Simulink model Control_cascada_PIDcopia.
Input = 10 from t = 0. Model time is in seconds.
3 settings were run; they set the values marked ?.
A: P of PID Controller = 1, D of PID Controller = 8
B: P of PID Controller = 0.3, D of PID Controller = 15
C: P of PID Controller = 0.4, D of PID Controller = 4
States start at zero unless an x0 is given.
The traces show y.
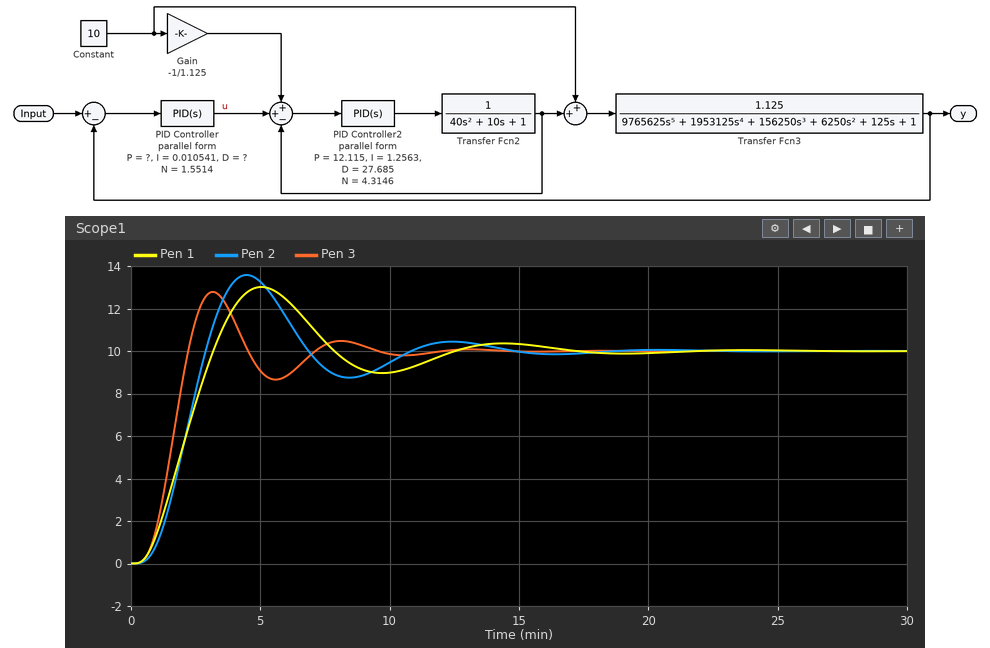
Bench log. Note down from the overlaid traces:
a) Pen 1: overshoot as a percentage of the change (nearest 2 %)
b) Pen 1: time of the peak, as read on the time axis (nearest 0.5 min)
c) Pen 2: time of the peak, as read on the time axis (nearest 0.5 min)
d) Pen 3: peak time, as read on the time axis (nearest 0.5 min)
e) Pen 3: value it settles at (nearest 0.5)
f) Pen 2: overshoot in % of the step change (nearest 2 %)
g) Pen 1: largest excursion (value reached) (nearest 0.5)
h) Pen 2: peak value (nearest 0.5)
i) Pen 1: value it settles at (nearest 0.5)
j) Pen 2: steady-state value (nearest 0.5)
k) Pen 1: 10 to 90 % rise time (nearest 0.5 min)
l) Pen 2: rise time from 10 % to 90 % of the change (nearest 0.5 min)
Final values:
30 %
5.0 min
4.5 min
3.0 min
10.0
36 %
13.0
13.5
10.0
10.0
2.0 min
1.5 min
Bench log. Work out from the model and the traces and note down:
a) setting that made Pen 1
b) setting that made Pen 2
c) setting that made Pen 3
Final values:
B
C
A
